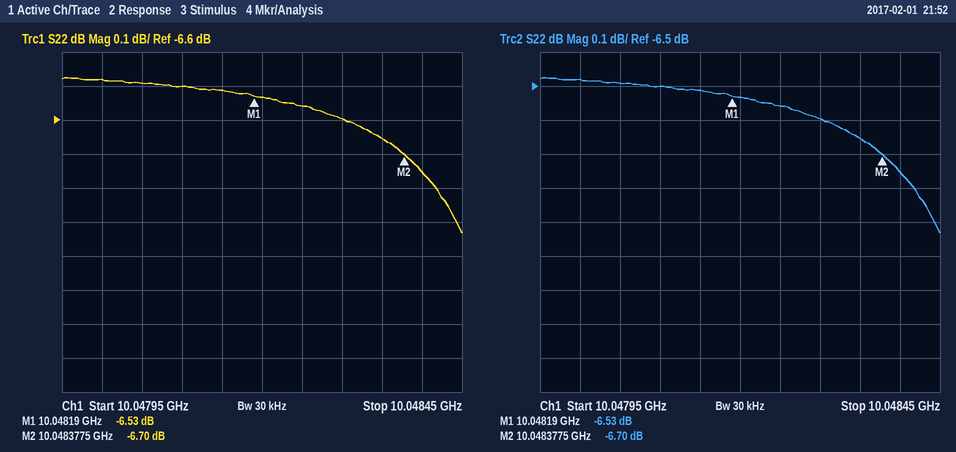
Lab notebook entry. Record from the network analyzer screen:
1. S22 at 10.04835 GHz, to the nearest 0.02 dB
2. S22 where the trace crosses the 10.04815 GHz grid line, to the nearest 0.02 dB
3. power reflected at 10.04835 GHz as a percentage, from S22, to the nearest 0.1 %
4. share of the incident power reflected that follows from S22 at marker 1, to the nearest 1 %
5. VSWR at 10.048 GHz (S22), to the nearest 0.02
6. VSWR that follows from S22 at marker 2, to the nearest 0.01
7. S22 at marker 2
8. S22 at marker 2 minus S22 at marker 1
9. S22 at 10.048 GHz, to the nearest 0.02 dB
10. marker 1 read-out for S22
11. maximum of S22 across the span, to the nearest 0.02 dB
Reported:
-6.66 dB
-6.52 dB
21.6 %
22 %
2.80
2.72
-6.70 dB
-0.17 dB
-6.48 dB
-6.53 dB
-6.48 dB
